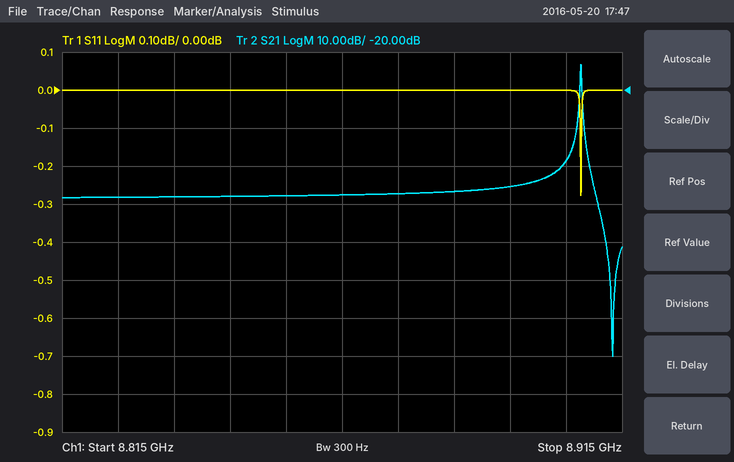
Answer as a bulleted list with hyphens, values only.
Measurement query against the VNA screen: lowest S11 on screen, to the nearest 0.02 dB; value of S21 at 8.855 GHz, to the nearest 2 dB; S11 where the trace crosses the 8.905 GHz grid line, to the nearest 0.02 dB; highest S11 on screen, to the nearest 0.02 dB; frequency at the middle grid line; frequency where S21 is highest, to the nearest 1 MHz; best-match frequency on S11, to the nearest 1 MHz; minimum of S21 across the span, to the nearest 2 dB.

- -0.28 dB
- -48 dB
- 0.00 dB
- 0.00 dB
- 8.865 GHz
- 8.908 GHz
- 8.908 GHz
- -90 dB
